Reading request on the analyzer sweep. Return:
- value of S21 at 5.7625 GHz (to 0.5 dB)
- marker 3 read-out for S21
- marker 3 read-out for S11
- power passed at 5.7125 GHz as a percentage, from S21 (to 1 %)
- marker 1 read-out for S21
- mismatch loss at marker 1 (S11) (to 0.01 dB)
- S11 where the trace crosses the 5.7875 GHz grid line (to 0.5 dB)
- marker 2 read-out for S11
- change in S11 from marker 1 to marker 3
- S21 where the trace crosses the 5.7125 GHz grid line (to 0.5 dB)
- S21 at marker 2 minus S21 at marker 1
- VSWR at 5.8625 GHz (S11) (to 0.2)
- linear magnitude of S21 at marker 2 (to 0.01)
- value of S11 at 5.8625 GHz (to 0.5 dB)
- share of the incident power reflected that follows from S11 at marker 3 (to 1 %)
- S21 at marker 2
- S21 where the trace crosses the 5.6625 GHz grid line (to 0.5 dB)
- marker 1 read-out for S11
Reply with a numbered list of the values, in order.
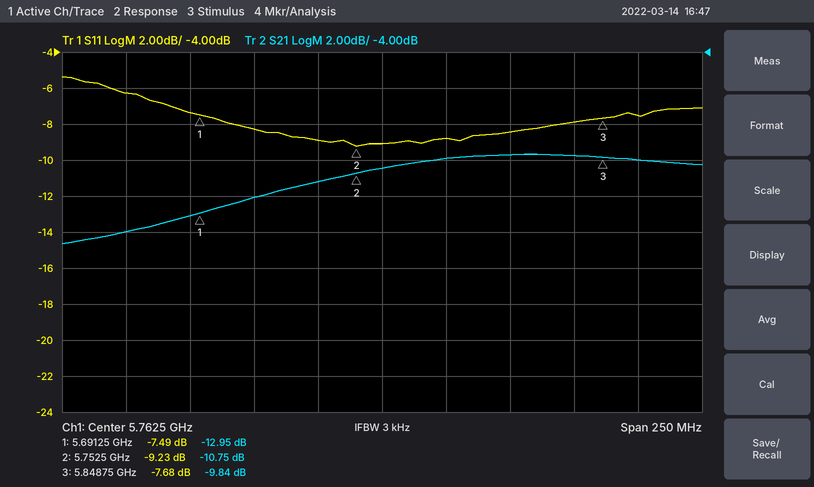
1. -10.5 dB
2. -9.84 dB
3. -7.68 dB
4. 6 %
5. -12.95 dB
6. 0.85 dB
7. -9.0 dB
8. -9.23 dB
9. -0.19 dB
10. -12.0 dB
11. 2.20 dB
12. 2.4
13. 0.29
14. -7.5 dB
15. 17 %
16. -10.75 dB
17. -14.0 dB
18. -7.49 dB
